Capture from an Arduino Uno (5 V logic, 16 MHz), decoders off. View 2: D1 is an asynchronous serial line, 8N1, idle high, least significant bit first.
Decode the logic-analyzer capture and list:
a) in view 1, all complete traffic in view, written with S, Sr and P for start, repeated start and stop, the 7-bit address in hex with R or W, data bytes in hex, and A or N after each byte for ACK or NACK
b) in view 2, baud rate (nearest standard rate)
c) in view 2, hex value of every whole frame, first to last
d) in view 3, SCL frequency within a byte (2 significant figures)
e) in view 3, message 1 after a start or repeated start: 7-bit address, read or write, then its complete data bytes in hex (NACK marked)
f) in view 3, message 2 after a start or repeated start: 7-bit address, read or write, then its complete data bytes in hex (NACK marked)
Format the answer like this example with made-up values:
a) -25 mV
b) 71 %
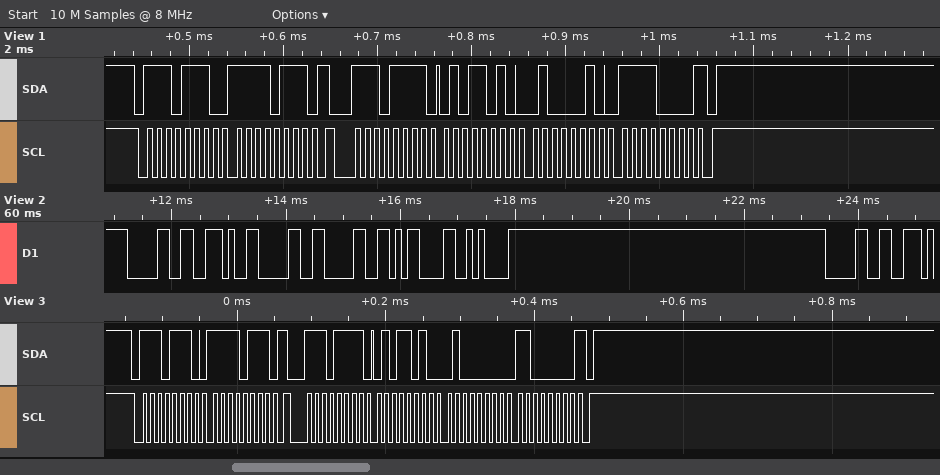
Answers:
a) S 77W A F7 A Sr 77R A 5A A 42 A F0 N P
b) 9600 baud
c) 30 2E 30 30 0D 0A 30
d) 100 kHz
e) 0x77 write: F7
f) 0x77 read: 5A 40 C0 NACK
